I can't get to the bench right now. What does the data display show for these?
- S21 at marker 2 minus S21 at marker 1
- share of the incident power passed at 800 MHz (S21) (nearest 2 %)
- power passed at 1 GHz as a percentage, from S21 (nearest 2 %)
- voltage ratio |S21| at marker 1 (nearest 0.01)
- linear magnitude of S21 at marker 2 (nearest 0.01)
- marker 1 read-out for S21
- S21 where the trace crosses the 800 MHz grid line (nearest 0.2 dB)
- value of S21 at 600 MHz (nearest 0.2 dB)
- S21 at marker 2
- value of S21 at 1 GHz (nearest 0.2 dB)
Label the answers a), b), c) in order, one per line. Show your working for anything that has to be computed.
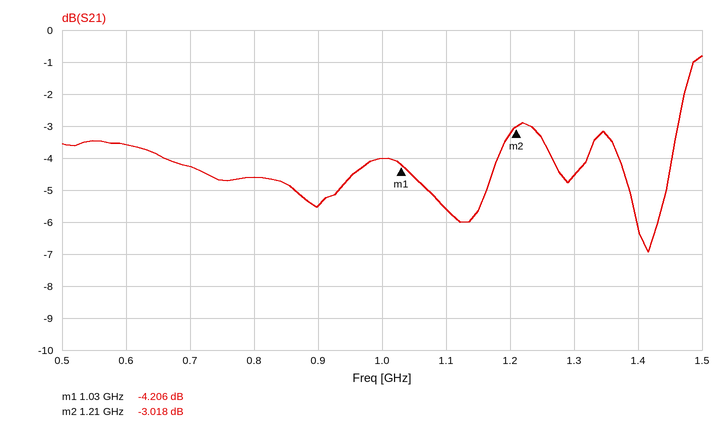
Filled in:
a) -3.018 − (-4.206) = 1.188 dB
b) 10^(-4.6/10) ≈ 34.7 %, so 34 % to the nearest 2 %
c) 10^(-4/10) ≈ 40 %
d) 10^(-4.206/20) ≈ 0.62
e) 10^(-3.018/20) ≈ 0.71
f) -4.206 dB
g) -4.6 dB
h) -3.6 dB
i) -3.018 dB
j) -4.0 dB
